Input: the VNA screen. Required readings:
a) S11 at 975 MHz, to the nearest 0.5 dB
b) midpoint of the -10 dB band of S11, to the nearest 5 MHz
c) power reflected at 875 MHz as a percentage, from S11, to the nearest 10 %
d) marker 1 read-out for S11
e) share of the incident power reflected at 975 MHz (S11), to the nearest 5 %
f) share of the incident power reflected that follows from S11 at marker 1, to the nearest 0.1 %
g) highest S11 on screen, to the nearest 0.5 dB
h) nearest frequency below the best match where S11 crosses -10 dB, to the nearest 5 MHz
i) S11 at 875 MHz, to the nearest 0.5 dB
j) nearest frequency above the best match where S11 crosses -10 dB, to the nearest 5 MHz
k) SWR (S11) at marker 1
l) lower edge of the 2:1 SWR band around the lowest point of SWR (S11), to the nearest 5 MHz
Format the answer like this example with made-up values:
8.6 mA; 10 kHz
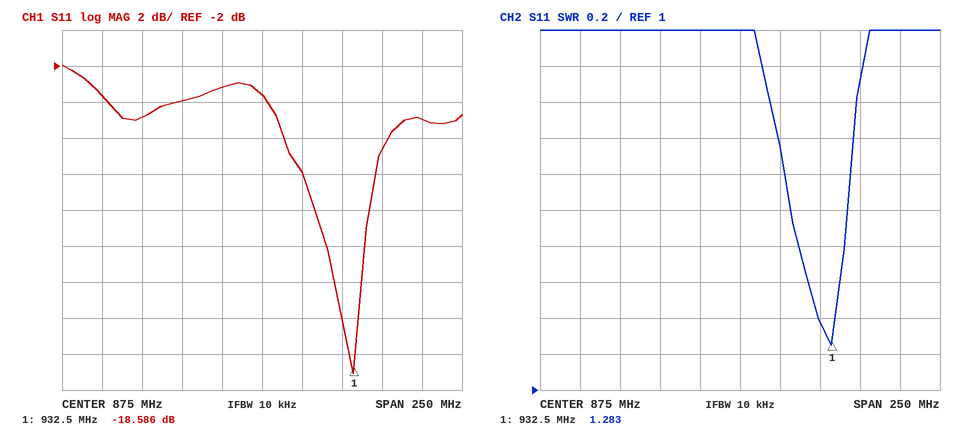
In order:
-5.0 dB; 925 MHz; 40 %; -18.586 dB; 30 %; 1.4 %; -2.0 dB; 910 MHz; -3.5 dB; 940 MHz; 1.283; 905 MHz
